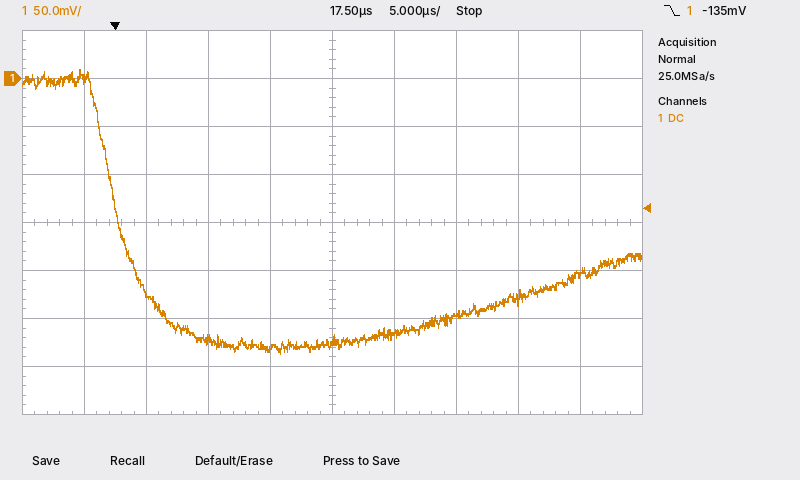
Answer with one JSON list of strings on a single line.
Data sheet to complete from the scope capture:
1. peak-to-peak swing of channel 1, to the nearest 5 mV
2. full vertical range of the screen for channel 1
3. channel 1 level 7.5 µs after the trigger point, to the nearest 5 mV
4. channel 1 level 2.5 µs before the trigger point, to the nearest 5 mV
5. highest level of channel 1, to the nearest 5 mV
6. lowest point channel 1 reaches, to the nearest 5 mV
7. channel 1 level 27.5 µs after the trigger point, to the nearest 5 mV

["295 mV", "400 mV", "-270 mV", "0 mV", "10 mV", "-285 mV", "-245 mV"]
